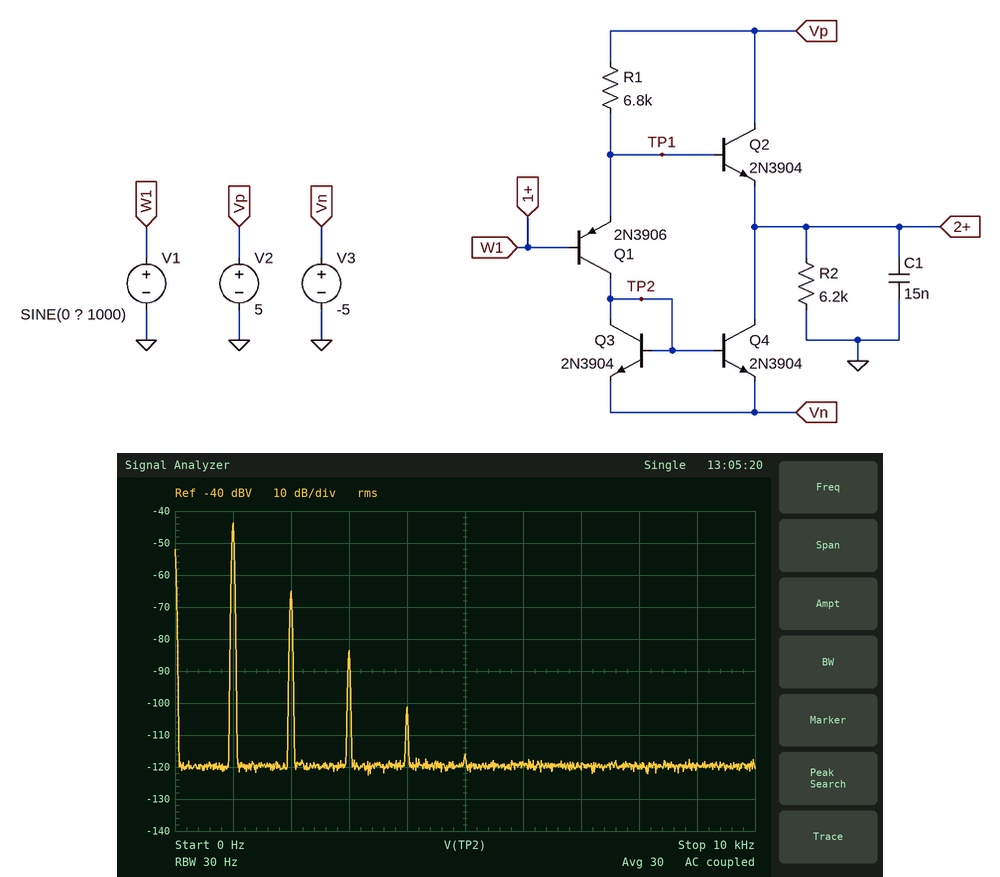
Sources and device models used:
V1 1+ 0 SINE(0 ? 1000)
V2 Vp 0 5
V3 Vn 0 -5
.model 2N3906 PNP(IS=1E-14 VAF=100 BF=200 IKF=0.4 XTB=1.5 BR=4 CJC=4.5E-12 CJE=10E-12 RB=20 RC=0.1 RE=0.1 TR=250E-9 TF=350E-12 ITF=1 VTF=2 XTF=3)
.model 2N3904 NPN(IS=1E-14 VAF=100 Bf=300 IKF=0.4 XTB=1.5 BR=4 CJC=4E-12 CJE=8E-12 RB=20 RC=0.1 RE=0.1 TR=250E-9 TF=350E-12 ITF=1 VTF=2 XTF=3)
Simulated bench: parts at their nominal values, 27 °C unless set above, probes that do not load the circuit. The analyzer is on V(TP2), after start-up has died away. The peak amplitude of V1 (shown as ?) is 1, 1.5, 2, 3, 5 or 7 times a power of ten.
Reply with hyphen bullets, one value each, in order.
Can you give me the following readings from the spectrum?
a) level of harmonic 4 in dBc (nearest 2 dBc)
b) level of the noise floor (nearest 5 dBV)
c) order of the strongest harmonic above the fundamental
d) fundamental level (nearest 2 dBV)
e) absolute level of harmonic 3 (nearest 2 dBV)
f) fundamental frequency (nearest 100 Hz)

- -58 dBc
- -120 dBV
- 2
- -44 dBV
- -84 dBV
- 1.0 kHz
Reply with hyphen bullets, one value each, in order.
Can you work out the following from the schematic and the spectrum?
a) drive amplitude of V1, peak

- 1.5 V
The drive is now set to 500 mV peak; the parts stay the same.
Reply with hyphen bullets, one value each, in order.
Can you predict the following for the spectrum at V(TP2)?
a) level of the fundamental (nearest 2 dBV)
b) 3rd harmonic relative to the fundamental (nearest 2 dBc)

- -54 dBV
- -60 dBc
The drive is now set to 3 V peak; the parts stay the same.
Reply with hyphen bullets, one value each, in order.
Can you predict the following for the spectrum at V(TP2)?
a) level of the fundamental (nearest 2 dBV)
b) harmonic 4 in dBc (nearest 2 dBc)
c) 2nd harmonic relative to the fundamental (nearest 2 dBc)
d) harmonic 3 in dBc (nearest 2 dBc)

- -36 dBV
- -36 dBc
- -14 dBc
- -26 dBc
